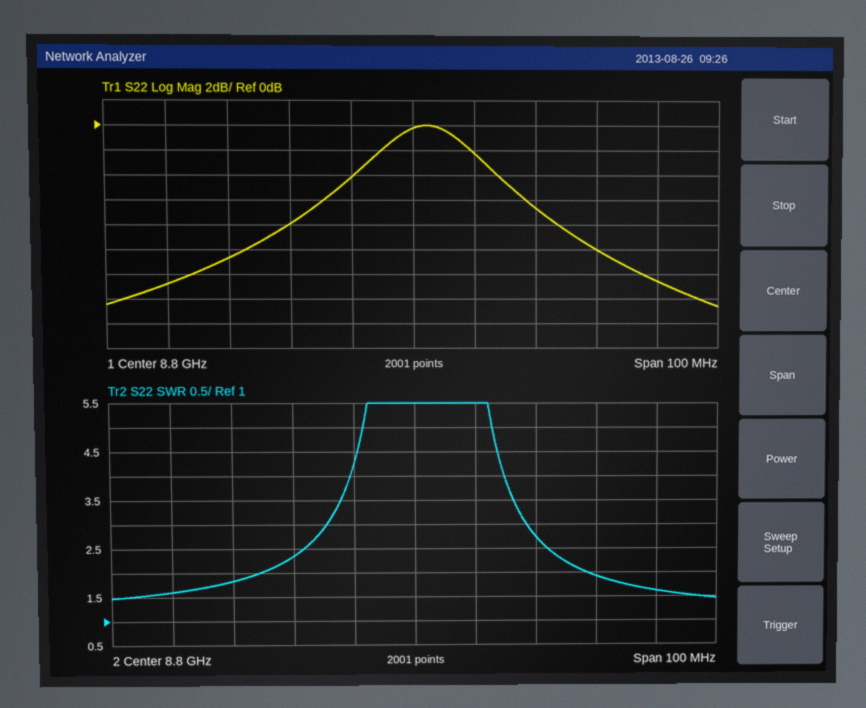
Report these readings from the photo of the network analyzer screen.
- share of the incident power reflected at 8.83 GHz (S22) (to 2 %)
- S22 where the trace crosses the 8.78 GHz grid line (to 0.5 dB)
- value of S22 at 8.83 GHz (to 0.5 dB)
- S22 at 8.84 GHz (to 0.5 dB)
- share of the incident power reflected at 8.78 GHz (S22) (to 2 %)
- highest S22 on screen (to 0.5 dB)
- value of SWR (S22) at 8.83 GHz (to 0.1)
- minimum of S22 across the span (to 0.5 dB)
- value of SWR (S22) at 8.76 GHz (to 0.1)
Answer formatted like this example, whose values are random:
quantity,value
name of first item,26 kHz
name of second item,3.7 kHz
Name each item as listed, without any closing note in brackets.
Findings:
quantity,value
share of the incident power reflected at 8.83 GHz (S22),10 %
S22 where the trace crosses the 8.78 GHz grid line,-8.0 dB
value of S22 at 8.83 GHz,-10.0 dB
S22 at 8.84 GHz,-12.5 dB
share of the incident power reflected at 8.78 GHz (S22),16 %
highest S22 on screen,0.0 dB
value of SWR (S22) at 8.83 GHz,1.9
minimum of S22 across the span,-14.5 dB
value of SWR (S22) at 8.76 GHz,1.6
